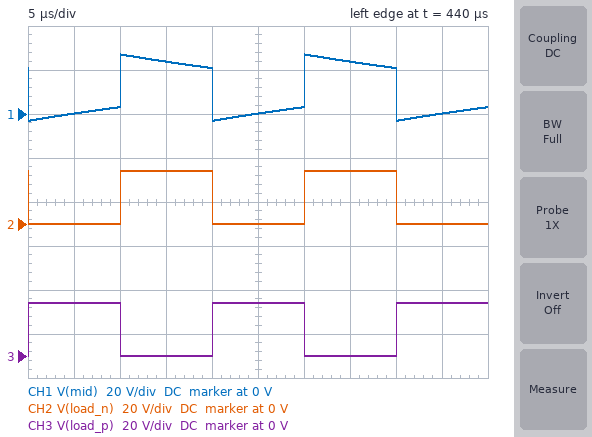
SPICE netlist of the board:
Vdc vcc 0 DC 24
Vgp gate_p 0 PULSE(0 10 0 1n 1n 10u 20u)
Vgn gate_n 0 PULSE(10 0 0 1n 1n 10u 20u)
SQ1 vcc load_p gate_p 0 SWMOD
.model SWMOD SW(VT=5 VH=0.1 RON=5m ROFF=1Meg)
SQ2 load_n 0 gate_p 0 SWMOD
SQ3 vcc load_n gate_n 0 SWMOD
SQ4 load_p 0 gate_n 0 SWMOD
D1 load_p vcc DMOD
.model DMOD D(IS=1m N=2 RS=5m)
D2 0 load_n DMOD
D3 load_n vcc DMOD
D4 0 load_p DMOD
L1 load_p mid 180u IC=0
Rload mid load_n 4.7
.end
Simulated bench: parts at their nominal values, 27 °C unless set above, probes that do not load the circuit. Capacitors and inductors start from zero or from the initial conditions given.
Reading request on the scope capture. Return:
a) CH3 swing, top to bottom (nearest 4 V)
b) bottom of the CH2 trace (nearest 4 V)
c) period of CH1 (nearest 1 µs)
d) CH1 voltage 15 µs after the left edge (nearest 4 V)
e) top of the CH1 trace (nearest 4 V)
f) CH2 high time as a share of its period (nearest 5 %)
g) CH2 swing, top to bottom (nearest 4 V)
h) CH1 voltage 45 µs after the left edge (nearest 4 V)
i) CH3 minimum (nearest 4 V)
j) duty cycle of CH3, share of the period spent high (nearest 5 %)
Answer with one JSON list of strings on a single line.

["24 V", "0 V", "20 µs", "24 V", "28 V", "50 %", "24 V", "0 V", "0 V", "50 %"]
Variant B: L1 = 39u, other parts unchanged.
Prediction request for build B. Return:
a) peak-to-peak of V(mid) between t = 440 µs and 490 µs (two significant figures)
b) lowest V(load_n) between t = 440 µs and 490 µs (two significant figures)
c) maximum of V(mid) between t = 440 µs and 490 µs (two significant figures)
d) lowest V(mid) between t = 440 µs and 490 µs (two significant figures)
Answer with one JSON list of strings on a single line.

["50 V", "-14 mV", "37 V", "-13 V"]
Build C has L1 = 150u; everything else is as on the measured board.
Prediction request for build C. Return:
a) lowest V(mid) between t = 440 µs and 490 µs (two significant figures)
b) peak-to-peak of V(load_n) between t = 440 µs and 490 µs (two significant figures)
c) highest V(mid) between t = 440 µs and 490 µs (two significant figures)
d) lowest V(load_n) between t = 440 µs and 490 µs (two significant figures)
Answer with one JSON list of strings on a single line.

["-3.7 V", "24 V", "28 V", "-4.0 mV"]
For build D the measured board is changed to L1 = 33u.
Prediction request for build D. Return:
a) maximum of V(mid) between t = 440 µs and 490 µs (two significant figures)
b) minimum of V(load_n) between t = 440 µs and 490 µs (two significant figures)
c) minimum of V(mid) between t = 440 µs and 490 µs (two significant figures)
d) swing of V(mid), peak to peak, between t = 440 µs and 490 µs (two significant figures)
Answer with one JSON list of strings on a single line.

["39 V", "-16 mV", "-15 V", "53 V"]
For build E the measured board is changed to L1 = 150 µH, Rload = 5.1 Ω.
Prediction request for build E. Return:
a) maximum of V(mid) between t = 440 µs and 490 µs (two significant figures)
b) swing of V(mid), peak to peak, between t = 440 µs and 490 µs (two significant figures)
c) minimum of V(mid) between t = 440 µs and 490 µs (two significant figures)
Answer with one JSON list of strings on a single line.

["28 V", "32 V", "-4.0 V"]
